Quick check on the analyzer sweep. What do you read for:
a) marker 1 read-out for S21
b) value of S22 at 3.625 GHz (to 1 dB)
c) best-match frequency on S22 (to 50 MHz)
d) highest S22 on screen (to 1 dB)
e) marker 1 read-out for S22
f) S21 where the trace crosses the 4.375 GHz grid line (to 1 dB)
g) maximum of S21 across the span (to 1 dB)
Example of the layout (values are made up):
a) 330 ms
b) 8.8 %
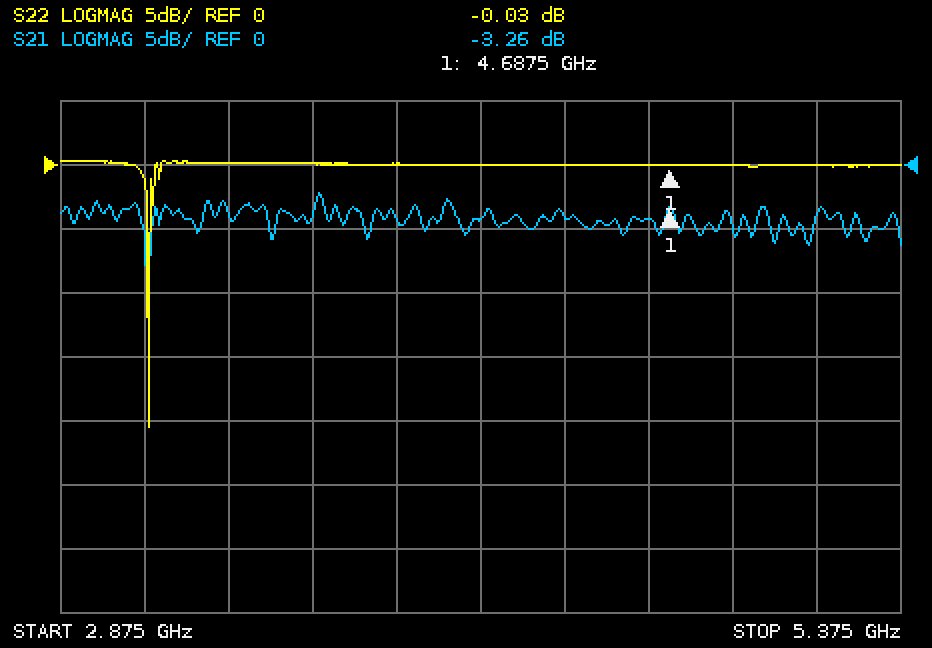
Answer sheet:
a) -3.26 dB
b) 0 dB
c) 3.15 GHz
d) 0 dB
e) -0.03 dB
f) -4 dB
g) -2 dB
